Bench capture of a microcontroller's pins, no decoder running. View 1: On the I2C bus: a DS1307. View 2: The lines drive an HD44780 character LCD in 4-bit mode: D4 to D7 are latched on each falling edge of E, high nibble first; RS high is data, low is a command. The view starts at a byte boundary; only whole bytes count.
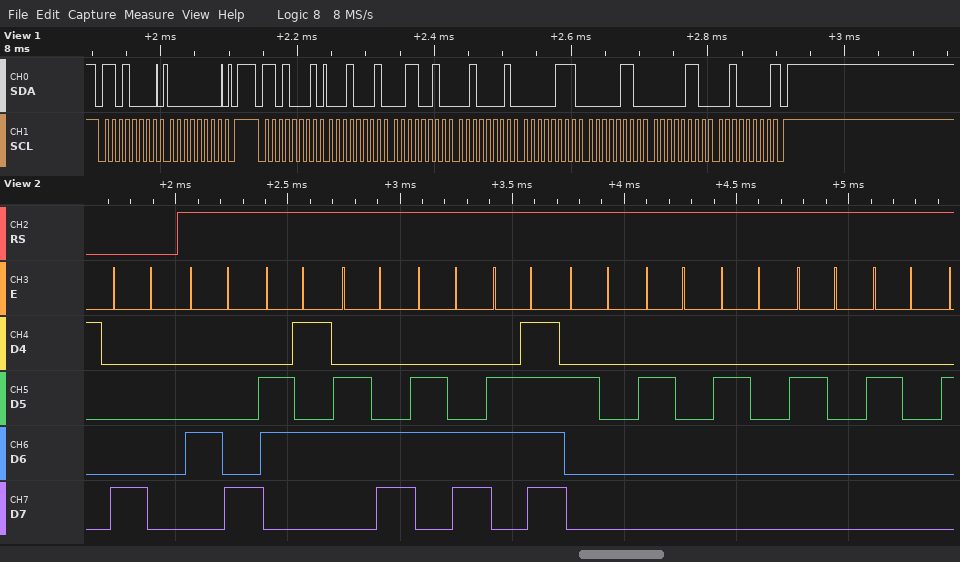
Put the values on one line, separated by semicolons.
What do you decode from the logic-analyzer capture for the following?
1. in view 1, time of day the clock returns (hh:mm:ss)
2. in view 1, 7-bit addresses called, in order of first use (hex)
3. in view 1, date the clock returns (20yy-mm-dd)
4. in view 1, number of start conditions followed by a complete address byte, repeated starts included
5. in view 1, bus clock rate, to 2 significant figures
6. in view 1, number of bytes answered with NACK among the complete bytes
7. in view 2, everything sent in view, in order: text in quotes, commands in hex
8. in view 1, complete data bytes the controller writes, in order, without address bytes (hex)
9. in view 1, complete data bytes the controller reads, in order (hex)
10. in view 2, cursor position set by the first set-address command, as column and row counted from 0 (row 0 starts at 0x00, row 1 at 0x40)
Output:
21:32:11; 0x68; 2020-06-06; 2; 100 kHz; 1; 0x80 "Hello     "; 00; 11 32 21 07 06 06 20; column 0, row 0
